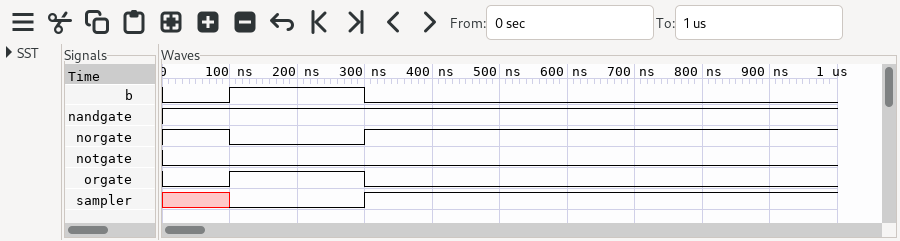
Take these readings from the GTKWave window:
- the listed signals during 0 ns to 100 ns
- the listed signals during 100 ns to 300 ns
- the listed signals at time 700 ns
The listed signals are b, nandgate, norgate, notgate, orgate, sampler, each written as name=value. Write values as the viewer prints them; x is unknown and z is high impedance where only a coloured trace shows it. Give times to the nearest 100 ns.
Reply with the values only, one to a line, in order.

b=0, nandgate=1, norgate=1, notgate=0, orgate=0, sampler=x
b=1, nandgate=1, norgate=0, notgate=0, orgate=1, sampler=0
b=0, nandgate=1, norgate=1, notgate=0, orgate=0, sampler=1
